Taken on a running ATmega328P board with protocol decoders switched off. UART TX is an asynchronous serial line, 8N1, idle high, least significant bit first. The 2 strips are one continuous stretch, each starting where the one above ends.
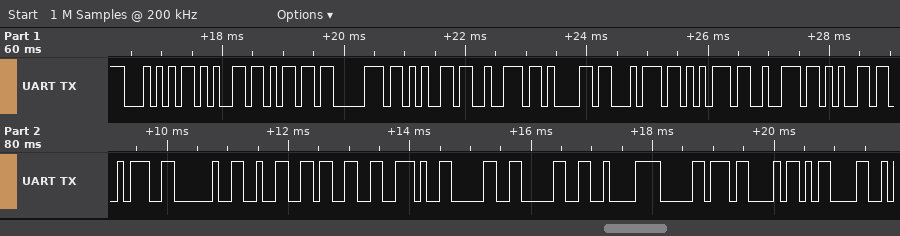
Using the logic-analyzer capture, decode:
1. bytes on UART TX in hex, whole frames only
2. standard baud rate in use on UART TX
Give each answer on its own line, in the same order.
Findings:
0x54 0x65 0x6D 0x70 0x65 0x72 0x61 0x74 0x75 0x72 0x65 0x3A 0x20 0x32 0x33 0x2E 0x30 0x30 0xC2 0xB0 0x43 0x0D
9600 baud
